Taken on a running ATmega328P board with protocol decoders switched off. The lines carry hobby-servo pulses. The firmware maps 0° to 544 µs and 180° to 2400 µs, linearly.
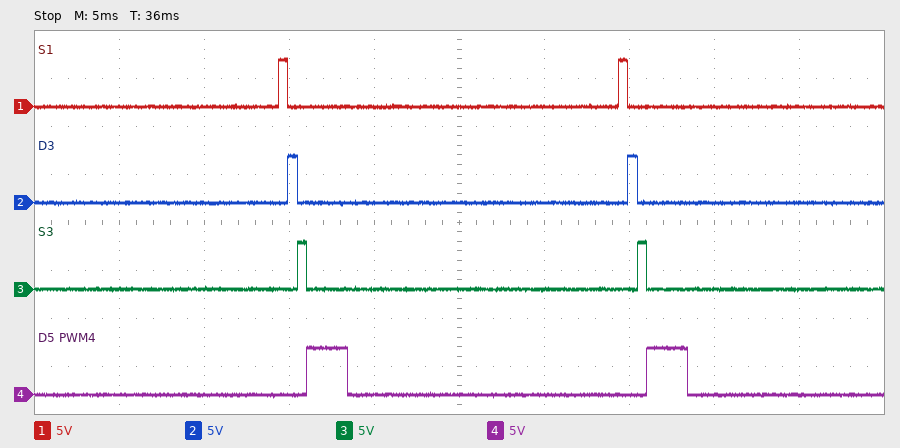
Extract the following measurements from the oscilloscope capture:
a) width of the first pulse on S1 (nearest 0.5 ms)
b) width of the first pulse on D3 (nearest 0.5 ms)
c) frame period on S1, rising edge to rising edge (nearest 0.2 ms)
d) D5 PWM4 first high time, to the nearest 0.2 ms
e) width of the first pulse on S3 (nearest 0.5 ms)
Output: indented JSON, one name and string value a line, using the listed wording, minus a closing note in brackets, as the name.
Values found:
{
  "width of the first pulse on S1": "0.5 ms",
  "width of the first pulse on D3": "0.5 ms",
  "frame period on S1, rising edge to rising edge": "20.0 ms",
  "D5 PWM4 first high time, to the nearest 0.2 ms": "2.4 ms",
  "width of the first pulse on S3": "0.5 ms"
}
